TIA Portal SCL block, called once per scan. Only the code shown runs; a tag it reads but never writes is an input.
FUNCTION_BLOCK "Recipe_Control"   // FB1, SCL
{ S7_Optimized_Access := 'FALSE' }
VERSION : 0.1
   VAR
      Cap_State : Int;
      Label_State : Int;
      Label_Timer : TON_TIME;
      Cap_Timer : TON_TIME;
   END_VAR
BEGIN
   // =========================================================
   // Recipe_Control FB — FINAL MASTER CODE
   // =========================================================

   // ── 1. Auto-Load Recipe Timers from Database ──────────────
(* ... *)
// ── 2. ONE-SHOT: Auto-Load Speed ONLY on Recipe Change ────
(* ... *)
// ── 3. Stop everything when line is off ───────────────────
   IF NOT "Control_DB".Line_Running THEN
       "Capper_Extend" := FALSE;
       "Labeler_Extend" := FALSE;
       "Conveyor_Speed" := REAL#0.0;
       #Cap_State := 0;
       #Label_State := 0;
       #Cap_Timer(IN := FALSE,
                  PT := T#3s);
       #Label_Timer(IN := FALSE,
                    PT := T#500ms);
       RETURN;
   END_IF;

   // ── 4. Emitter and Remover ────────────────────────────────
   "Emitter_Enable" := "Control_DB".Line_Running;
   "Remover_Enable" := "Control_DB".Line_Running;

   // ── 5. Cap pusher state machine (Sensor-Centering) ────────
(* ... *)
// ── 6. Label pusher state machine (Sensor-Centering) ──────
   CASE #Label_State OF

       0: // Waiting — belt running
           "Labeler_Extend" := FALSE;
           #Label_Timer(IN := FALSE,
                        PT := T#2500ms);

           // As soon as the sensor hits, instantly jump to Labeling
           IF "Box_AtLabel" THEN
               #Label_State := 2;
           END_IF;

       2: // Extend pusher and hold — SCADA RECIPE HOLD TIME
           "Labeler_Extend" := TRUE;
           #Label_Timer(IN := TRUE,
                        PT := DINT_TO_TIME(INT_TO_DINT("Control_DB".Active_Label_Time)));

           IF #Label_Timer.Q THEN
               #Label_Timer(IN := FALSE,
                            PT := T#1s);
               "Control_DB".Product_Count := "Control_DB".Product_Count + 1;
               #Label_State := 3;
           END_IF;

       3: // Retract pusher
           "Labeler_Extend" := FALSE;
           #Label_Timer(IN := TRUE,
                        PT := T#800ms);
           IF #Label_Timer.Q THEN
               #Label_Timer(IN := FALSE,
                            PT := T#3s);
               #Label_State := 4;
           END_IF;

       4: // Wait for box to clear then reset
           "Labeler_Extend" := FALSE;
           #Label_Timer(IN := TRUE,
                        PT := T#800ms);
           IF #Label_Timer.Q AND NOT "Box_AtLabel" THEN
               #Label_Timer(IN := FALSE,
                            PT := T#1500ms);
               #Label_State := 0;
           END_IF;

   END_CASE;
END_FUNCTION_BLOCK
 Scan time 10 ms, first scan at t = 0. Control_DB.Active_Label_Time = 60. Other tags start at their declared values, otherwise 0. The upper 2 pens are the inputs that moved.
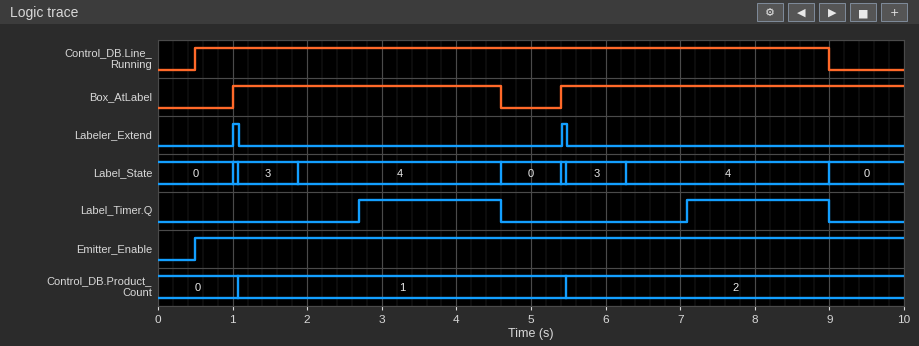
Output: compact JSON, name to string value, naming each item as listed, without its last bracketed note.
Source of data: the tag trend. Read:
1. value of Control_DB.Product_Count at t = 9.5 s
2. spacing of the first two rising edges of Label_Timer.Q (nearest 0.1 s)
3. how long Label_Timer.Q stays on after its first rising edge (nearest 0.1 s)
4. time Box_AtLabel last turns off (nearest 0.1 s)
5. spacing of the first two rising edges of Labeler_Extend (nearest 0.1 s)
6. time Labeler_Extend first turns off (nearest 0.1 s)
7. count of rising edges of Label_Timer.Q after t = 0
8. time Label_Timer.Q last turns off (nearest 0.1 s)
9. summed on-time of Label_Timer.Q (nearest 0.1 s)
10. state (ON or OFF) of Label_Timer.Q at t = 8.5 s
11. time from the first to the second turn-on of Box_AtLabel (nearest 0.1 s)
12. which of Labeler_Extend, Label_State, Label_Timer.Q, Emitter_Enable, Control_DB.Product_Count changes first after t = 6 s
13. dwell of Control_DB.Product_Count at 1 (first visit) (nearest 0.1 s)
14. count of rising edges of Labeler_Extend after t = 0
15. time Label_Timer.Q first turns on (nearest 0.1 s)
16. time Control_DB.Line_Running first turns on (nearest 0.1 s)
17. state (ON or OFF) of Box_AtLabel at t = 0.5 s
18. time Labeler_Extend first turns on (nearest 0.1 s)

{"value of Control_DB.Product_Count at t = 9.5 s": "2", "spacing of the first two rising edges of Label_Timer.Q": "4.4 s", "how long Label_Timer.Q stays on after its first rising edge": "1.9 s", "time Box_AtLabel last turns off": "4.6 s", "spacing of the first two rising edges of Labeler_Extend": "4.4 s", "time Labeler_Extend first turns off": "1.1 s", "count of rising edges of Label_Timer.Q after t = 0": "2", "time Label_Timer.Q last turns off": "9.0 s", "summed on-time of Label_Timer.Q": "3.8 s", "state (ON or OFF) of Label_Timer.Q at t = 8.5 s": "ON", "time from the first to the second turn-on of Box_AtLabel": "4.4 s", "which of Labeler_Extend, Label_State, Label_Timer.Q, Emitter_Enable, Control_DB.Product_Count changes first after t = 6 s": "Label_State", "dwell of Control_DB.Product_Count at 1 (first visit)": "4.4 s", "count of rising edges of Labeler_Extend after t = 0": "2", "time Label_Timer.Q first turns on": "2.7 s", "time Control_DB.Line_Running first turns on": "0.5 s", "state (ON or OFF) of Box_AtLabel at t = 0.5 s": "OFF", "time Labeler_Extend first turns on": "1.0 s"}
